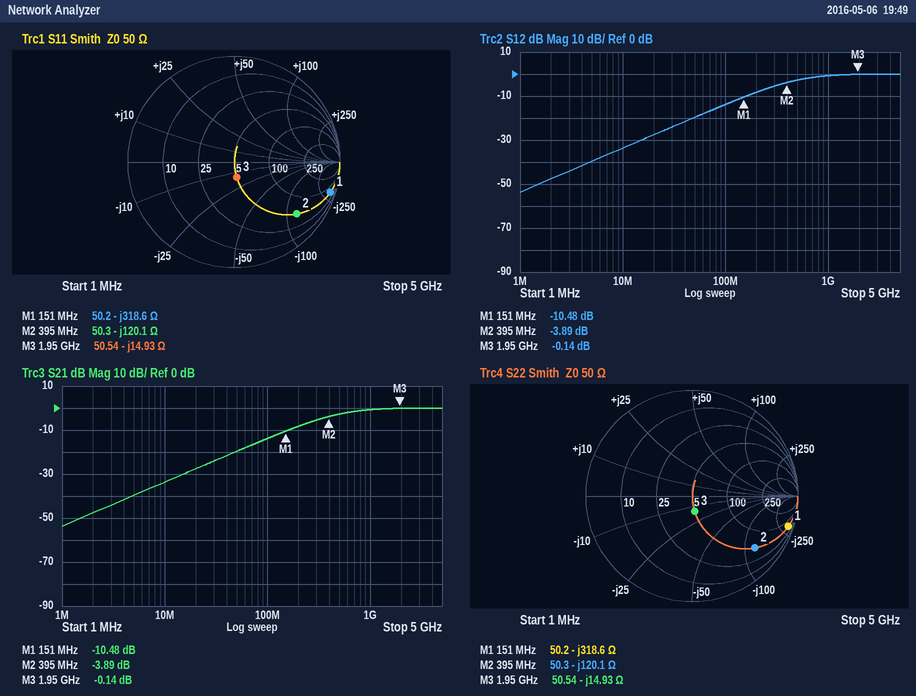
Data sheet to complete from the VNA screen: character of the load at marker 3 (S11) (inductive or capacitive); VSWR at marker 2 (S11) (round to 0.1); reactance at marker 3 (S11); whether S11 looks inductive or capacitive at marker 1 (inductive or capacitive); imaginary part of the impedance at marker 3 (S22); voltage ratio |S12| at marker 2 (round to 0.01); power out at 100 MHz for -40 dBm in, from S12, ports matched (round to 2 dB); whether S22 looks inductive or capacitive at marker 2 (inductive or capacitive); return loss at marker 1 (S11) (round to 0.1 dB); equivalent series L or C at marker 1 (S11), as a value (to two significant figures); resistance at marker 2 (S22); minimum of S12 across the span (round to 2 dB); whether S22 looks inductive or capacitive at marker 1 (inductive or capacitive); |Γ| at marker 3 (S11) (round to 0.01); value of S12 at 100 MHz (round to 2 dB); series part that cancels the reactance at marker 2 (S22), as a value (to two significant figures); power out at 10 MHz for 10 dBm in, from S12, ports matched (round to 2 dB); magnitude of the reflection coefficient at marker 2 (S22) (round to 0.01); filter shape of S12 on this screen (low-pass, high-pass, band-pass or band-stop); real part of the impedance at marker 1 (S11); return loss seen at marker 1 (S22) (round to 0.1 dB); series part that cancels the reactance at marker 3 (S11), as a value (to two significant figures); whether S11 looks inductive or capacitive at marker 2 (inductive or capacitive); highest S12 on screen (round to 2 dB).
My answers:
capacitive
7.6
-14.93 Ω
capacitive
-14.93 Ω
0.64
-54 dBm
capacitive
0.4 dB
3.3 pF
50.3 Ω
-54 dB
capacitive
0.15
-14 dB
48 nH
-24 dBm
0.77
high-pass
50.2 Ω
0.4 dB
1.2 nH
capacitive
0 dB
